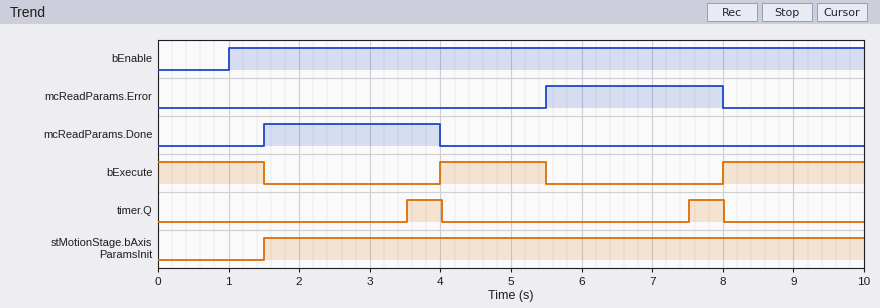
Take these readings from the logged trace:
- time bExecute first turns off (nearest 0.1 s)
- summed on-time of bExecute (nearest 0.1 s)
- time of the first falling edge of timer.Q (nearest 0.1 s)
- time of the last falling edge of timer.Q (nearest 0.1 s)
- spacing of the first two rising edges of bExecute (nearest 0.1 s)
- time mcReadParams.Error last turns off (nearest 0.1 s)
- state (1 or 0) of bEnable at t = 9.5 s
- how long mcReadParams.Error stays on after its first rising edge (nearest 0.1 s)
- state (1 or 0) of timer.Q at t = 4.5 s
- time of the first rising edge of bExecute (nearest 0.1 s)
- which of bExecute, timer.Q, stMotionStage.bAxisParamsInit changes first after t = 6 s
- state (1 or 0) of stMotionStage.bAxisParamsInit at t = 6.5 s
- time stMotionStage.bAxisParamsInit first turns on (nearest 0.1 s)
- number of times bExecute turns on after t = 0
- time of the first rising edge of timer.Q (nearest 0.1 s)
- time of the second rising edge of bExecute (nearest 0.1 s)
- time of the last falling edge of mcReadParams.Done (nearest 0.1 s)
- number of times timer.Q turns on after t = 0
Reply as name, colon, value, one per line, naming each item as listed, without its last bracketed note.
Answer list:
time bExecute first turns off: 1.5 s
summed on-time of bExecute: 5.0 s
time of the first falling edge of timer.Q: 4.0 s
time of the last falling edge of timer.Q: 8.0 s
spacing of the first two rising edges of bExecute: 4.0 s
time mcReadParams.Error last turns off: 8.0 s
state (1 or 0) of bEnable at t = 9.5 s: 1
how long mcReadParams.Error stays on after its first rising edge: 2.5 s
state (1 or 0) of timer.Q at t = 4.5 s: 0
time of the first rising edge of bExecute: 4.0 s
which of bExecute, timer.Q, stMotionStage.bAxisParamsInit changes first after t = 6 s: timer.Q
state (1 or 0) of stMotionStage.bAxisParamsInit at t = 6.5 s: 1
time stMotionStage.bAxisParamsInit first turns on: 1.5 s
number of times bExecute turns on after t = 0: 2
time of the first rising edge of timer.Q: 3.5 s
time of the second rising edge of bExecute: 8.0 s
time of the last falling edge of mcReadParams.Done: 4.0 s
number of times timer.Q turns on after t = 0: 2
